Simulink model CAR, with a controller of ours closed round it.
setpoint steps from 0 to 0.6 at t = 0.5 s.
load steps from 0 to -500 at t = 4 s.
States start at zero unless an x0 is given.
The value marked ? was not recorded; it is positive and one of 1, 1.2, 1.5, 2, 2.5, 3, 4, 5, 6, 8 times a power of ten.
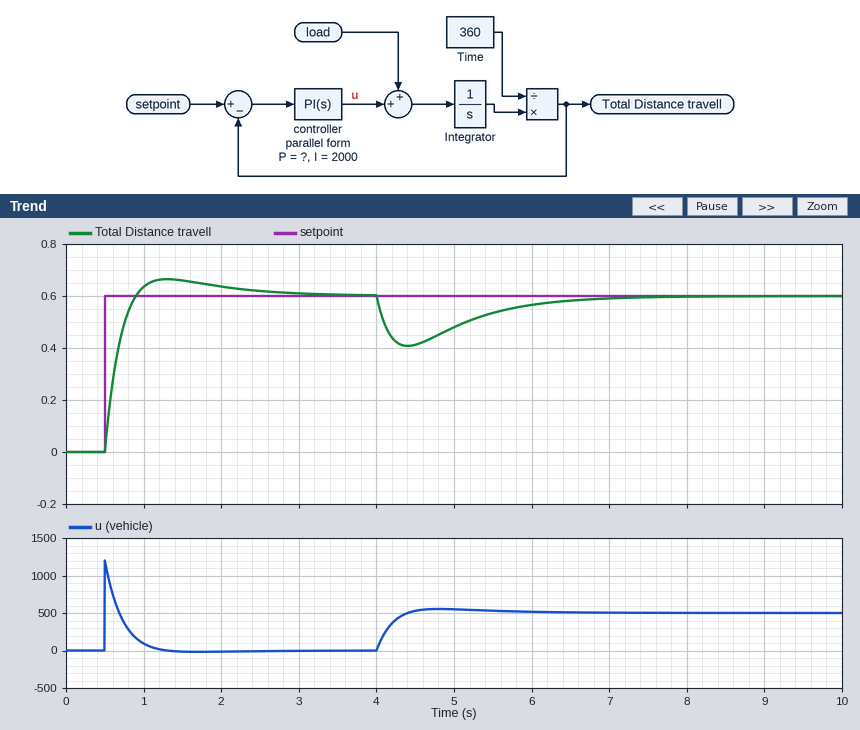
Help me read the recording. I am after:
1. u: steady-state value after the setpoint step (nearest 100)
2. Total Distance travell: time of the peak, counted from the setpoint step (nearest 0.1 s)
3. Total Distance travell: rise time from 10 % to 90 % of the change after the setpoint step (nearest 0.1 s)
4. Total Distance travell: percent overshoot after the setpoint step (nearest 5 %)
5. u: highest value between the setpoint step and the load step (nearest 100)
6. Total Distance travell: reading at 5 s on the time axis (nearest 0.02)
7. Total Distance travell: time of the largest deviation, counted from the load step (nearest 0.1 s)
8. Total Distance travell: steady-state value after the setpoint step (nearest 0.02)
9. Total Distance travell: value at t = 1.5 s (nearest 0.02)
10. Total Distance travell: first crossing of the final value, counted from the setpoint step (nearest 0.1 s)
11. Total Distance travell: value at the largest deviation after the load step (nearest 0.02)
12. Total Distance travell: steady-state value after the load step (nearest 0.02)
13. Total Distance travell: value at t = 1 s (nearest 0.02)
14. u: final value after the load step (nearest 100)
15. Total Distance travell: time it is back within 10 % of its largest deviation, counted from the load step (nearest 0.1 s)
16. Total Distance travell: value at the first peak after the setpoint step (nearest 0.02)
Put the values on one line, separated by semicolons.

0; 0.8 s; 0.3 s; 10 %; 1200; 0.48; 0.4 s; 0.60; 0.66; 0.4 s; 0.40; 0.60; 0.64; 500; 2.4 s; 0.66
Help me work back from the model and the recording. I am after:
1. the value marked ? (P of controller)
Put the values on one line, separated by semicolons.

2000
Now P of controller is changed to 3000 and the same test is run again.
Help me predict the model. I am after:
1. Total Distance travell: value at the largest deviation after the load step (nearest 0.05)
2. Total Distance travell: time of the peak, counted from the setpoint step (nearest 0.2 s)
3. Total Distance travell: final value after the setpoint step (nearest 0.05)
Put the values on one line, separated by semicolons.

0.45; 0.6 s; 0.60
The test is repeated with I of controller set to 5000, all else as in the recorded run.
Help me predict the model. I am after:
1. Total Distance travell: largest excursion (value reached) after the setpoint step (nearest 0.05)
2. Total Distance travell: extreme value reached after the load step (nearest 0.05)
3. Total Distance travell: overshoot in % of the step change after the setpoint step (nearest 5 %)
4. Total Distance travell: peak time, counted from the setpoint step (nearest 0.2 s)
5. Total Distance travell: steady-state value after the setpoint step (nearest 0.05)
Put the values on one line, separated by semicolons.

0.70; 0.45; 20 %; 0.6 s; 0.60
